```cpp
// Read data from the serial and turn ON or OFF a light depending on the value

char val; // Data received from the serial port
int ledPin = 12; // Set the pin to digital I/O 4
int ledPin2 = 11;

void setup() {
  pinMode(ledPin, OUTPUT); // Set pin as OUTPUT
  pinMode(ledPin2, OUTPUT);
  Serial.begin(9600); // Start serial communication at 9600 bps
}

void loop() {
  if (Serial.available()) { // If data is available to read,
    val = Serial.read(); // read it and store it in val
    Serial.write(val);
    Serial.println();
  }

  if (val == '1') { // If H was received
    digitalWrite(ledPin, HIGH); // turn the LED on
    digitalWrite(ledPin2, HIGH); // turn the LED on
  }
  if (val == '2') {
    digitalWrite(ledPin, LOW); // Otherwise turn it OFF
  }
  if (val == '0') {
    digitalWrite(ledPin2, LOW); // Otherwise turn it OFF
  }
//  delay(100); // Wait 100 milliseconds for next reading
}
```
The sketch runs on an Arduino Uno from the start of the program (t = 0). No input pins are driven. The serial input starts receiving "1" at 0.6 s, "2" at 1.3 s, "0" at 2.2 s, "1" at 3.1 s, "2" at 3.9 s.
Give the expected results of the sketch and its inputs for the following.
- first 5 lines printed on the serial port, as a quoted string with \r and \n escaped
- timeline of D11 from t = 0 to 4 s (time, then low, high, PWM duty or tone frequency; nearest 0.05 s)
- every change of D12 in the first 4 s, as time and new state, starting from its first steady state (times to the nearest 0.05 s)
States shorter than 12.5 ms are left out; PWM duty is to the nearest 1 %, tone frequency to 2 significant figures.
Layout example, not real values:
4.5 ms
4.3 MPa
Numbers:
"1\r\n2\r\n0\r\n1\r\n2\r\n"
0 s low; 0.6 s high; 2.2 s low; 3.1 s high
0 s low; 0.6 s high; 1.3 s low; 3.1 s high; 3.9 s low
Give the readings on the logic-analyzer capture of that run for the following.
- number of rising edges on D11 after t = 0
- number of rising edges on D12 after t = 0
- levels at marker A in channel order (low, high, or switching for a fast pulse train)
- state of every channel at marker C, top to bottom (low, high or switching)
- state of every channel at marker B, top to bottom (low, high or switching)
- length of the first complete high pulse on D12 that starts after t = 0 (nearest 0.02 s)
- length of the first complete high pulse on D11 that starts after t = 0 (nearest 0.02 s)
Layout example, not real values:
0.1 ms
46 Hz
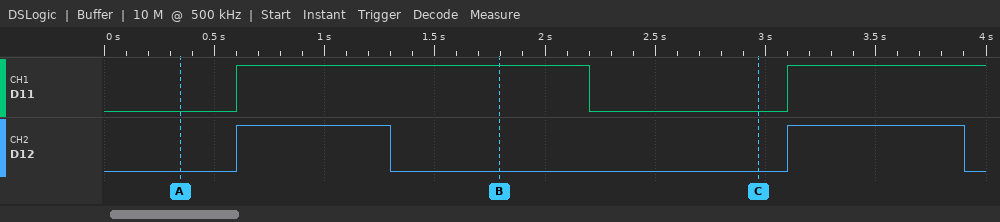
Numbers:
2
2
D11 low, D12 low
D11 low, D12 low
D11 high, D12 low
0.70 s
1.60 s
